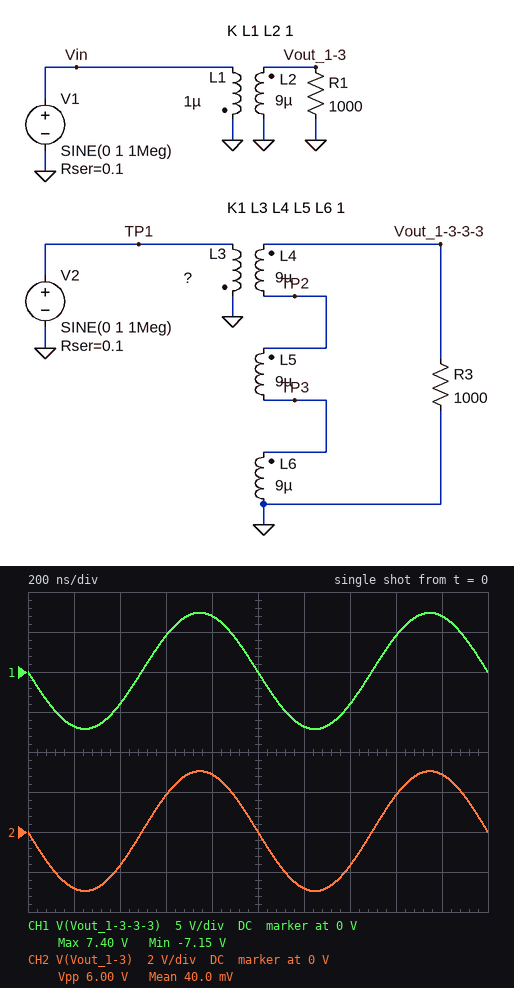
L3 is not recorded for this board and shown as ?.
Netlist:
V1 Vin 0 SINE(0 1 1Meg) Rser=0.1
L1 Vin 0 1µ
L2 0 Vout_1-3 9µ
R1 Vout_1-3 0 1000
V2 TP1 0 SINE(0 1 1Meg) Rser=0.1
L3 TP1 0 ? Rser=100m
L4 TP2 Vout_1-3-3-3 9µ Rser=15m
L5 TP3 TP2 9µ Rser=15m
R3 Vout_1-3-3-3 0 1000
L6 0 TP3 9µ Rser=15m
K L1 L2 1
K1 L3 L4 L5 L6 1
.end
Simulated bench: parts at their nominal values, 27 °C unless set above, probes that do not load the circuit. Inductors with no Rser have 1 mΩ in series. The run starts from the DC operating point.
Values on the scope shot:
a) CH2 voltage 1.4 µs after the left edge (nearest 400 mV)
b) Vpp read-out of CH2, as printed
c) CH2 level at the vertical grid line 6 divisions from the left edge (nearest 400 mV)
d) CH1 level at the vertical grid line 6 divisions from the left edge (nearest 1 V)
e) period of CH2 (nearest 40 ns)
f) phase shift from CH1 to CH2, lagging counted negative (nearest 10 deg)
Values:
-1.6 V
6.00 V
-2.8 V
-7 V
1.00 µs
0 deg
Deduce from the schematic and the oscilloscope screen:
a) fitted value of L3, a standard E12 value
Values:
1.5 µH
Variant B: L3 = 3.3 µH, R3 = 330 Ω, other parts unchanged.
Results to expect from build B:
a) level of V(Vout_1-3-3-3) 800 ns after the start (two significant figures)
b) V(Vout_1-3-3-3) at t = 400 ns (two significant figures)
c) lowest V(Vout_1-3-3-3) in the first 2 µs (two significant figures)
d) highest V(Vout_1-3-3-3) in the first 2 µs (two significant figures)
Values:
4.7 V
-2.8 V
-4.8 V
4.9 V
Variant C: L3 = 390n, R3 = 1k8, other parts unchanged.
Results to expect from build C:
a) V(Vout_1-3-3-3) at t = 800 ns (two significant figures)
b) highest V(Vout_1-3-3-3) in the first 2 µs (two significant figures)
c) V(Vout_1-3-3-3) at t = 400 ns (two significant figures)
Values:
14 V
15 V
-6.4 V
